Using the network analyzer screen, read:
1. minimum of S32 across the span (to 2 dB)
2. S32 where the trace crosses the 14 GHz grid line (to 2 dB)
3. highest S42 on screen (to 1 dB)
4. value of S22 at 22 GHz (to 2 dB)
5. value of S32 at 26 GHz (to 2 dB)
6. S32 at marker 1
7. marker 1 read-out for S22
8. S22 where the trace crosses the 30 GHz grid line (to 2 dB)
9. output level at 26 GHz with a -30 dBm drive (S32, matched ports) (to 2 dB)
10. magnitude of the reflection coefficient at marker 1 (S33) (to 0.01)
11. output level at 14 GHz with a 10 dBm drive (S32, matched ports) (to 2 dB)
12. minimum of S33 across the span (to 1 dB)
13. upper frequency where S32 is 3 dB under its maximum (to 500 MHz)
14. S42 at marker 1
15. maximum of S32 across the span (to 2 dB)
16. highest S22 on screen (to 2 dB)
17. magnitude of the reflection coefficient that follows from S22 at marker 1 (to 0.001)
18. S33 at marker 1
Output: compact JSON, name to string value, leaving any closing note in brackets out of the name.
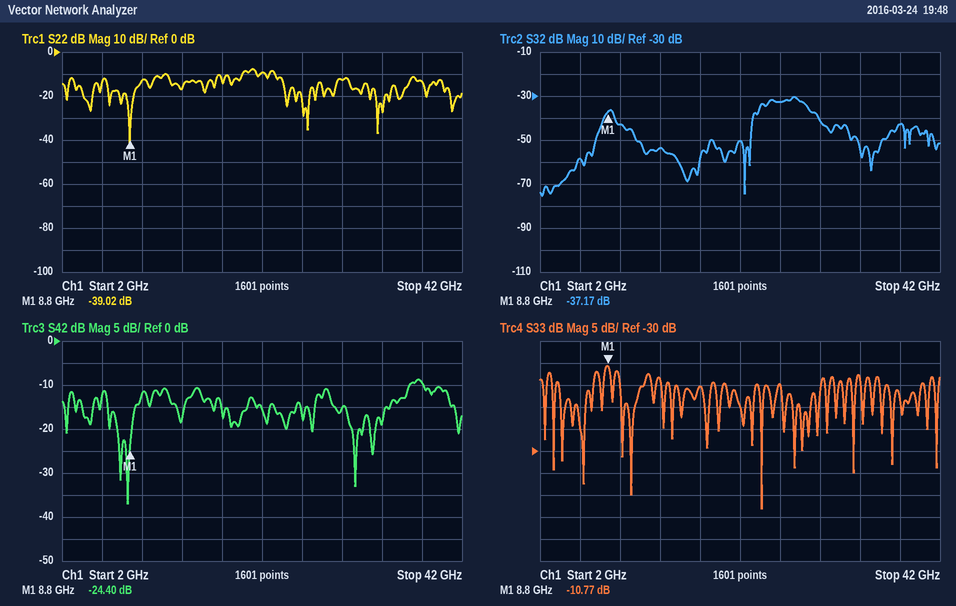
{"minimum of S32 across the span": "-76 dB", "S32 where the trace crosses the 14 GHz grid line": "-54 dB", "highest S42 on screen": "-9 dB", "value of S22 at 22 GHz": "-10 dB", "value of S32 at 26 GHz": "-32 dB", "S32 at marker 1": "-37.17 dB", "marker 1 read-out for S22": "-39.02 dB", "S22 where the trace crosses the 30 GHz grid line": "-12 dB", "output level at 26 GHz with a -30 dBm drive (S32, matched ports)": "-62 dBm", "magnitude of the reflection coefficient at marker 1 (S33)": "0.29", "output level at 14 GHz with a 10 dBm drive (S32, matched ports)": "-44 dBm", "minimum of S33 across the span": "-43 dB", "upper frequency where S32 is 3 dB under its maximum": "28.5 GHz", "S42 at marker 1": "-24.40 dB", "maximum of S32 across the span": "-30 dB", "highest S22 on screen": "-8 dB", "magnitude of the reflection coefficient that follows from S22 at marker 1": "0.011", "S33 at marker 1": "-10.77 dB"}
